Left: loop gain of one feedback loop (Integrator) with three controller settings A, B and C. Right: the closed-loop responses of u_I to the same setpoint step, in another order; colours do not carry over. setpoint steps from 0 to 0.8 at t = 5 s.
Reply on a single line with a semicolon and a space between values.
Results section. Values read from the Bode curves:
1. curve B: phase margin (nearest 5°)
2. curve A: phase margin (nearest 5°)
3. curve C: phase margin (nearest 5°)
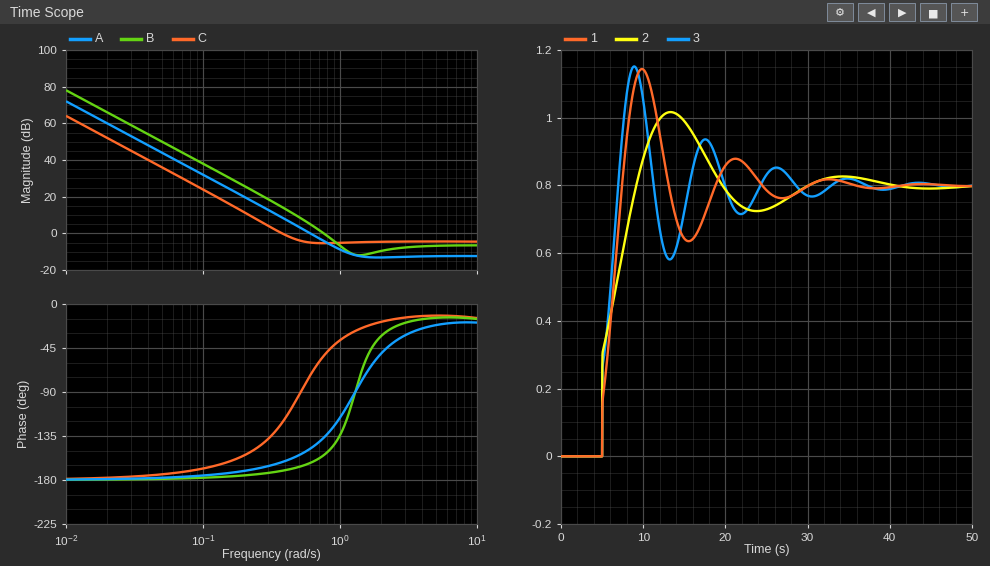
25°; 30°; 60°
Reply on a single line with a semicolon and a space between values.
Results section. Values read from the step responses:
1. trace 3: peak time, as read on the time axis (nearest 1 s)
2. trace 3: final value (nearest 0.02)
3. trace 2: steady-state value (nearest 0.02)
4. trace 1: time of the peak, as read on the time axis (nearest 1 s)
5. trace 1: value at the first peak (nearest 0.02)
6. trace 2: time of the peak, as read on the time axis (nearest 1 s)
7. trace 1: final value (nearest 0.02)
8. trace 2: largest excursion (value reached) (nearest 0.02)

9 s; 0.80; 0.80; 10 s; 1.14; 13 s; 0.80; 1.02
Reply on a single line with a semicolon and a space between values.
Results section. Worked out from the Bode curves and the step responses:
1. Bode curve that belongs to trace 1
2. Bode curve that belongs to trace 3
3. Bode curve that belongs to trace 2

A; B; C
